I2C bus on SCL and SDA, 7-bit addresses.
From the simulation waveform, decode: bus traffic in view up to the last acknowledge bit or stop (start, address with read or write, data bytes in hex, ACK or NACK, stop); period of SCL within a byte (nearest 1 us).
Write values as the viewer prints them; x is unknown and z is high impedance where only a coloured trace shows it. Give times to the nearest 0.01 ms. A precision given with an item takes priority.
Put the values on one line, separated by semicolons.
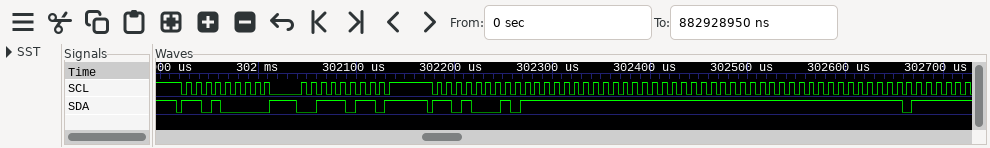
start, address 68 write ACK, 3B ACK, repeated start, address 68 read ACK, FF NACK, FF NACK, FF NACK, FF NACK, EF NACK; 10 us
